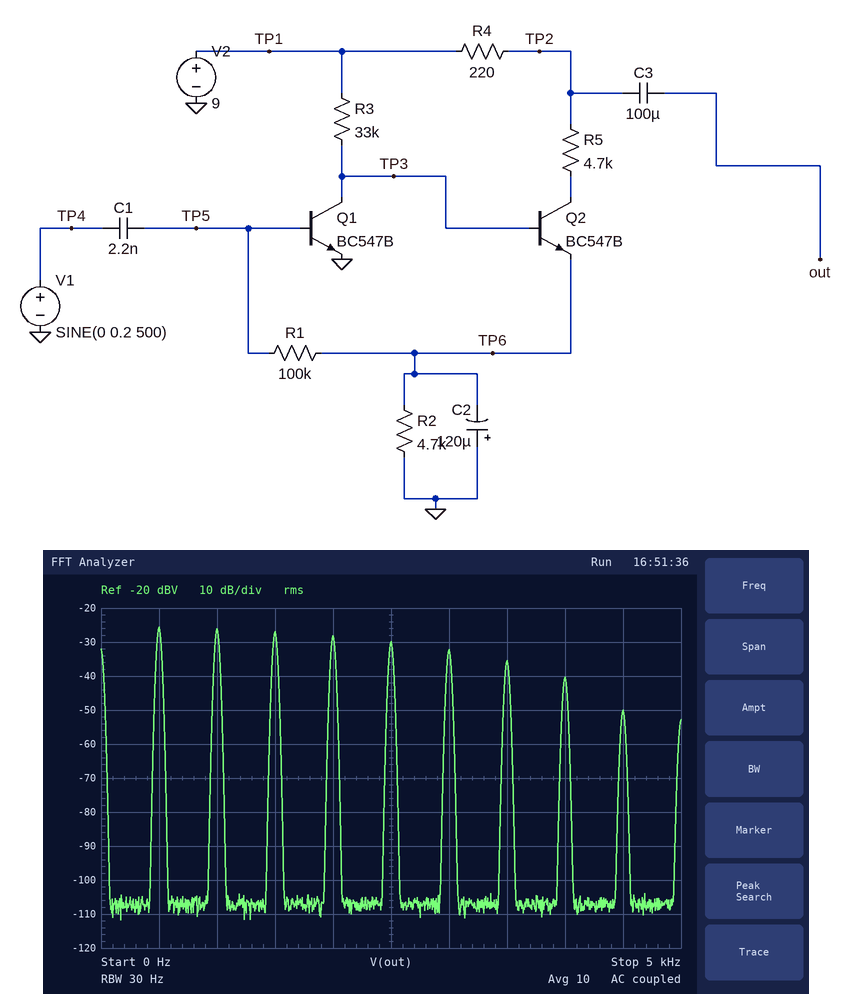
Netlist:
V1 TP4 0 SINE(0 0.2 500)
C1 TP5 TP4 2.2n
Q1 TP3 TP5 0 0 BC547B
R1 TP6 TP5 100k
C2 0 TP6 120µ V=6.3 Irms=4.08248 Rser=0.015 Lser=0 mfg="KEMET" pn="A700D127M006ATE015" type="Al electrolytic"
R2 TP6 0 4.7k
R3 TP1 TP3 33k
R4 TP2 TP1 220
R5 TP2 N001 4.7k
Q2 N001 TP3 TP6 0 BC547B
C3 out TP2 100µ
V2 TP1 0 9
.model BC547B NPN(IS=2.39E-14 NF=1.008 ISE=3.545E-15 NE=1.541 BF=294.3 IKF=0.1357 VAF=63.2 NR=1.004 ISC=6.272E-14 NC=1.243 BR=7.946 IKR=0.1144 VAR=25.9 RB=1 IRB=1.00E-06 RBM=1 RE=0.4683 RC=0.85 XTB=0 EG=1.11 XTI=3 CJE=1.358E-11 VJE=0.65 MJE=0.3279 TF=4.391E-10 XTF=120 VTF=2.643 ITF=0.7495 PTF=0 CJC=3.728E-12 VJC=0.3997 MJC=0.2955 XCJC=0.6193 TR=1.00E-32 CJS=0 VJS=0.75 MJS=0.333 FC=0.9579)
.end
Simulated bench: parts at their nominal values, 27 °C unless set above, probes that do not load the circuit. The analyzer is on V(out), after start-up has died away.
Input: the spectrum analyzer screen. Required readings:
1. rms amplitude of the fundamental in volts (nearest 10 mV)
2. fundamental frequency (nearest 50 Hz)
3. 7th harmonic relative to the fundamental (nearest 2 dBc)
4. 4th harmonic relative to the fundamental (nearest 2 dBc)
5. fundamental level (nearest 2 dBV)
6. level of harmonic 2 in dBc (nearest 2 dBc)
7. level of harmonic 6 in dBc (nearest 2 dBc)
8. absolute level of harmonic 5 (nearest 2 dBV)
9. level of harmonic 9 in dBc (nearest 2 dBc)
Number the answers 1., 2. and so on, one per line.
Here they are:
1. 50 mV
2. 500 Hz
3. -10 dBc
4. -2 dBc
5. -26 dBV
6. 0 dBc
7. -6 dBc
8. -30 dBV
9. -24 dBc
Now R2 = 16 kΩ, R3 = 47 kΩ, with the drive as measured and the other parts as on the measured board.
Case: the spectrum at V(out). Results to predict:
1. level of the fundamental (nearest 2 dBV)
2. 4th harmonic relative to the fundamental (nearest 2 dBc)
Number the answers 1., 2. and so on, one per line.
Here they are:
1. -36 dBV
2. 0 dBc
